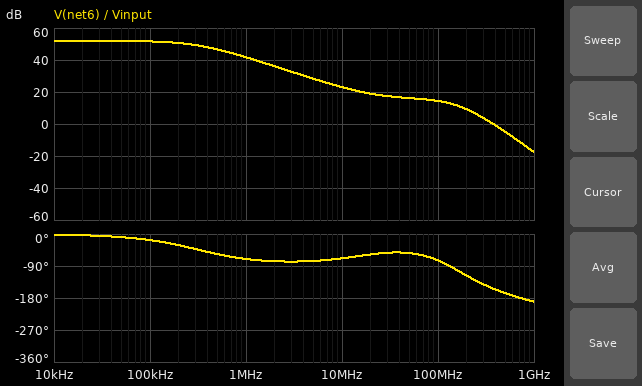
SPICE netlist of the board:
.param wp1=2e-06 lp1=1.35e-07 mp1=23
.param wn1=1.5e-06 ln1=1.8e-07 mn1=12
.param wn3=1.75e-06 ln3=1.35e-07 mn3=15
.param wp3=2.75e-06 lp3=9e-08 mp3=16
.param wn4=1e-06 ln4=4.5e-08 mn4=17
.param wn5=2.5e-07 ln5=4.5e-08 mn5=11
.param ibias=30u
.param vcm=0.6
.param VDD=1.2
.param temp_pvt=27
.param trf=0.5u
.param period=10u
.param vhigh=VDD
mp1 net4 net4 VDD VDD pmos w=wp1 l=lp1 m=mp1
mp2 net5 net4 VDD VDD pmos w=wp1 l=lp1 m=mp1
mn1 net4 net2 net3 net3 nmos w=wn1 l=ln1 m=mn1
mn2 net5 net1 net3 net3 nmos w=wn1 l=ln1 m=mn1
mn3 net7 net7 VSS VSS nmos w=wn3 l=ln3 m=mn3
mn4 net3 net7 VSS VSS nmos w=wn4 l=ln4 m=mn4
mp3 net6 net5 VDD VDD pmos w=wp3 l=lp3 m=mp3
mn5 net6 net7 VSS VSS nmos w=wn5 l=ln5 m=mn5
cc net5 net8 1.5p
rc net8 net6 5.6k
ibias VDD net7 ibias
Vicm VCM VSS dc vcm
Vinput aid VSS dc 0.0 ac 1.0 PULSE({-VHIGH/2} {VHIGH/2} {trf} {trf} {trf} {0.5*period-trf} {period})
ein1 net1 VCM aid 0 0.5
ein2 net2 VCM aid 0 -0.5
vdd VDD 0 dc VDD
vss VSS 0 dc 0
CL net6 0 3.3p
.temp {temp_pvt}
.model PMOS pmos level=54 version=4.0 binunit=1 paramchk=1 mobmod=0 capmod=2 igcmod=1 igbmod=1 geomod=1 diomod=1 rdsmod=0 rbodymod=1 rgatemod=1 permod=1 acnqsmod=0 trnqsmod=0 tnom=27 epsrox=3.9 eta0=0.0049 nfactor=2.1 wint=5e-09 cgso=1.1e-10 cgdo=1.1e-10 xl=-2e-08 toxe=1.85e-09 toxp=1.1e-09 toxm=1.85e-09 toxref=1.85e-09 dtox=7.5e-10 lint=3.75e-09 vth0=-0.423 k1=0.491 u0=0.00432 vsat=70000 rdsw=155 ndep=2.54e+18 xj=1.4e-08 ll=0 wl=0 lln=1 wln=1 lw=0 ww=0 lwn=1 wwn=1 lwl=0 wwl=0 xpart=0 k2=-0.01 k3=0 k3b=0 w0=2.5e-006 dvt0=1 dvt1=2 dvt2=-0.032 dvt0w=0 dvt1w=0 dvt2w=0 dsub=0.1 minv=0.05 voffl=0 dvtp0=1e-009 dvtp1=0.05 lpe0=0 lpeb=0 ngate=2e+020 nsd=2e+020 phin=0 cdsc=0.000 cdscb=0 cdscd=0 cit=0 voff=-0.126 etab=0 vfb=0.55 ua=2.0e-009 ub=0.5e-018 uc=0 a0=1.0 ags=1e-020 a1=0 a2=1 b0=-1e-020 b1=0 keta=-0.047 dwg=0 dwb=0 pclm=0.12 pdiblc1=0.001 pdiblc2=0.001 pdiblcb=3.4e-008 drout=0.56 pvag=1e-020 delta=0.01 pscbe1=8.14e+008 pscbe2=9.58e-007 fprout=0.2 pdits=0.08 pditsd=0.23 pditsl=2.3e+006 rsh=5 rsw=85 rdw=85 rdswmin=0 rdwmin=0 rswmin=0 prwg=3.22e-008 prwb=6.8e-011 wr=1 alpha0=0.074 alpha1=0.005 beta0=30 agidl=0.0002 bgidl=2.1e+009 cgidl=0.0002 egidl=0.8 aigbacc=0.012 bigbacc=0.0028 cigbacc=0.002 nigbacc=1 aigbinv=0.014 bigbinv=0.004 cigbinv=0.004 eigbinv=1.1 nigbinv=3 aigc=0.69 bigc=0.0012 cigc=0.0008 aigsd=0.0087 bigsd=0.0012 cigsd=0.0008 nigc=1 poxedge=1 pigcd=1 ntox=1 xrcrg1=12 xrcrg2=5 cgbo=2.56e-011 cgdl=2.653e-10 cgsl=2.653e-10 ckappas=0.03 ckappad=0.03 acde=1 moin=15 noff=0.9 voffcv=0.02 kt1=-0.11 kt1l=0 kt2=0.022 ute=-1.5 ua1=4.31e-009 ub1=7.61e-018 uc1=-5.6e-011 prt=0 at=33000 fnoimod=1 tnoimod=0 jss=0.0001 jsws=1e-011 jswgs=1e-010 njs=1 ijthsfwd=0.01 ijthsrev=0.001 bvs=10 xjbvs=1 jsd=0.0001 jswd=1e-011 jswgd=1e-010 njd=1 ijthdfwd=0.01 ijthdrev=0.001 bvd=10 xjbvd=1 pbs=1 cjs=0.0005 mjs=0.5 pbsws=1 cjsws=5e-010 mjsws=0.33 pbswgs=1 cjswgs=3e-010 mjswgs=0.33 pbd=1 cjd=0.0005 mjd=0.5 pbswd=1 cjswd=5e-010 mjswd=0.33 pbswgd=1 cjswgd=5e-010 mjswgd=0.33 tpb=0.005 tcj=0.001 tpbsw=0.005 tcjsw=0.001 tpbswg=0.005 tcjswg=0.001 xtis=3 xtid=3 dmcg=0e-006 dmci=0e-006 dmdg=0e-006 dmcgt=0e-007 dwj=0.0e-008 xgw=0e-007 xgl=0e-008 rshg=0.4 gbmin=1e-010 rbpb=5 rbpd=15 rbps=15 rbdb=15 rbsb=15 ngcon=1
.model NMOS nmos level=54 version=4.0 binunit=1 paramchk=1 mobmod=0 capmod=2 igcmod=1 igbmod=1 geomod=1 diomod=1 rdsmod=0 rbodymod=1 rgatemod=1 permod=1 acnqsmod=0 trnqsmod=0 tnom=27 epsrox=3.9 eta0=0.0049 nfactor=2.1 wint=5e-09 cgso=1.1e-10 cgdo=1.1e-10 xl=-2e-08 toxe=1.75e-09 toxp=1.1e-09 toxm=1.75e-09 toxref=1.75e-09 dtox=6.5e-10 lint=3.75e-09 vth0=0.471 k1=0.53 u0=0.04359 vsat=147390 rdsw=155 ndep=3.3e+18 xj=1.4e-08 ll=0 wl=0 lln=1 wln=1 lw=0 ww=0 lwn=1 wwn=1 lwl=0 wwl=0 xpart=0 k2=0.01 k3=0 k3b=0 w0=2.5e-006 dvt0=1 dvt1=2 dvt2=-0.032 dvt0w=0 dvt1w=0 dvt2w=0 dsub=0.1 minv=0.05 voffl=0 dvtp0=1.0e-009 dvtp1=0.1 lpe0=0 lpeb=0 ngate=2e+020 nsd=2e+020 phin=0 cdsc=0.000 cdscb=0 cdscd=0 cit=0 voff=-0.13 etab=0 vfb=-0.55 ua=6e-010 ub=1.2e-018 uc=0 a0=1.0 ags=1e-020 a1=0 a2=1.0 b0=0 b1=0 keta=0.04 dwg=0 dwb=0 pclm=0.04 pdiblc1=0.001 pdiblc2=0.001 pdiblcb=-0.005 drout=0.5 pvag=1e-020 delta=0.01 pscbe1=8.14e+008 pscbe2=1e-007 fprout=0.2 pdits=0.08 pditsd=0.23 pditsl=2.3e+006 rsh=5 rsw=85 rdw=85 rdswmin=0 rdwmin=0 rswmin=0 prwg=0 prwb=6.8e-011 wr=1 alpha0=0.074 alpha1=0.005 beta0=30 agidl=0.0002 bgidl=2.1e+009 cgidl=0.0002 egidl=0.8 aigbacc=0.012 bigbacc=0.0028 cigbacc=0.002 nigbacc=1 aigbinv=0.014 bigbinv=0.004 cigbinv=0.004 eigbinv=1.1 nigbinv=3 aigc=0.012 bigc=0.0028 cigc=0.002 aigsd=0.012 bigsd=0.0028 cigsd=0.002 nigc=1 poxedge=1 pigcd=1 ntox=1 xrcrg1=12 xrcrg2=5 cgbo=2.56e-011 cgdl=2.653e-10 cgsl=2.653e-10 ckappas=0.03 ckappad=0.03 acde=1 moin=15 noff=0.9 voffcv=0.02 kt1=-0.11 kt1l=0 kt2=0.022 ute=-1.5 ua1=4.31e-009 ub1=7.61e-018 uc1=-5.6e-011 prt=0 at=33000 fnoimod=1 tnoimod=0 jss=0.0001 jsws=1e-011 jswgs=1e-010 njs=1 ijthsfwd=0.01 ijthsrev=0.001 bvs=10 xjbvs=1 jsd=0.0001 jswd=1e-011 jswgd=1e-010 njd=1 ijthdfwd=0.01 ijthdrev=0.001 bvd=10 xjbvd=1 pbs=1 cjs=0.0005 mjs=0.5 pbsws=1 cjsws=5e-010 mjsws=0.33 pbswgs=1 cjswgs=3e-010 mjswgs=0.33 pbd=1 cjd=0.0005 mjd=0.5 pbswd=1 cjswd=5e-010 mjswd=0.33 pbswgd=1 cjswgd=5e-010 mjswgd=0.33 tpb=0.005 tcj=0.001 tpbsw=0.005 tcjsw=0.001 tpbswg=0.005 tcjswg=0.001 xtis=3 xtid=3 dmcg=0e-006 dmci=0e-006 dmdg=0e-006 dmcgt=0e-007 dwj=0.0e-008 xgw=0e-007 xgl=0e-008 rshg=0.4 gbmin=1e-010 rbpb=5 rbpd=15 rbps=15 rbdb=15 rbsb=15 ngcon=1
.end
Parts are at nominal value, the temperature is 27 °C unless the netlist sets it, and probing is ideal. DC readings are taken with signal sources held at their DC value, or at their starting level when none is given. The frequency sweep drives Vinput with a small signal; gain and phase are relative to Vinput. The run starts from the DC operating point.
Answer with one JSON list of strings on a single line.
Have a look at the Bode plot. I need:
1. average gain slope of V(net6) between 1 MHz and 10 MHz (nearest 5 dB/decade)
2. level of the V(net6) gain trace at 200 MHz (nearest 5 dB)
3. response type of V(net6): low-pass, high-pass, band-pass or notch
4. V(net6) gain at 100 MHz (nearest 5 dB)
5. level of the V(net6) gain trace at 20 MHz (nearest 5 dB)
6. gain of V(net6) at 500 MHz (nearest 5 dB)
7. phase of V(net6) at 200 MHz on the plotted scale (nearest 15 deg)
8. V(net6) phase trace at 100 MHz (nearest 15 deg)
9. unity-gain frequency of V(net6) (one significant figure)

["-20 dB/decade", "10 dB", "low-pass", "15 dB", "20 dB", "-5 dB", "-120 deg", "-75 deg", "400 MHz"]
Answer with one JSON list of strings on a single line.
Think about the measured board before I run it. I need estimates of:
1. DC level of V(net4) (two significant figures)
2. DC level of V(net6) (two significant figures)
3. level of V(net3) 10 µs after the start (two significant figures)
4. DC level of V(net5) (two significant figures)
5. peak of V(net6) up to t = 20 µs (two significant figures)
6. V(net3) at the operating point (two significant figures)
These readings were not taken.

["710 mV", "740 mV", "350 mV", "710 mV", "1.2 V", "140 mV"]
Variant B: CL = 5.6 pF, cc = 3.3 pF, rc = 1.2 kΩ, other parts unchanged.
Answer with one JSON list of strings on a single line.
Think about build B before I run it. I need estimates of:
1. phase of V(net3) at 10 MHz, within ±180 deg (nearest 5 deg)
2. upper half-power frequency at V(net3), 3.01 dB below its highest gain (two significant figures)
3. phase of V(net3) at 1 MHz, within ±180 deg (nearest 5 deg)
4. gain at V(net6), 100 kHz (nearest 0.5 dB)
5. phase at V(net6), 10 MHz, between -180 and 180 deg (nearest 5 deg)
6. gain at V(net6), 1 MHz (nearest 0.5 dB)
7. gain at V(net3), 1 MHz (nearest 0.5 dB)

["140 deg", "150 kHz", "105 deg", "50.5 dB", "-90 deg", "35.5 dB", "-32.5 dB"]
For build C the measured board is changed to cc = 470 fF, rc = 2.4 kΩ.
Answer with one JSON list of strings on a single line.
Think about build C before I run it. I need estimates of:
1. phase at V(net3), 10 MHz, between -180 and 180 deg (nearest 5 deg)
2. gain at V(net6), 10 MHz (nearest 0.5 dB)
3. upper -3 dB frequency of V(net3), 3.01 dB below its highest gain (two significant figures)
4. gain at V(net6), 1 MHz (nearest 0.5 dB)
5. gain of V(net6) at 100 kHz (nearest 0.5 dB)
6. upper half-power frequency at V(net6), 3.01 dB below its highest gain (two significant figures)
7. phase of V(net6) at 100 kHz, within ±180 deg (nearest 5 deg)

["130 deg", "31.5 dB", "960 kHz", "49.0 dB", "52.0 dB", "950 kHz", "-5 deg"]
